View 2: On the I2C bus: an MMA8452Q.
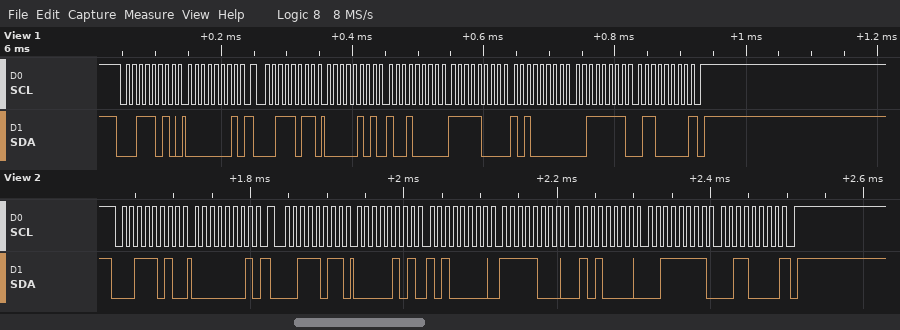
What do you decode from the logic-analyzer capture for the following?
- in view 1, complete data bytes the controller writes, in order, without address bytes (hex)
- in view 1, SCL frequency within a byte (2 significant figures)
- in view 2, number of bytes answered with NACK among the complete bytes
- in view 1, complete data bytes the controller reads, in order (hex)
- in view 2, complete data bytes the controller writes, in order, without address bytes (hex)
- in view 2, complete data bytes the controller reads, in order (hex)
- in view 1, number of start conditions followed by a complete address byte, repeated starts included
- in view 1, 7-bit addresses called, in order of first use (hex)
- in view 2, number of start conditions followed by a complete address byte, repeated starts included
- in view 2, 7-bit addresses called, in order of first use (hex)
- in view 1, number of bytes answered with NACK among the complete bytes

01
100 kHz
1
05 90 F8 A0 3F 60
01
05 A0 F8 50 3F 30
2
0x1D
2
0x1D
1
